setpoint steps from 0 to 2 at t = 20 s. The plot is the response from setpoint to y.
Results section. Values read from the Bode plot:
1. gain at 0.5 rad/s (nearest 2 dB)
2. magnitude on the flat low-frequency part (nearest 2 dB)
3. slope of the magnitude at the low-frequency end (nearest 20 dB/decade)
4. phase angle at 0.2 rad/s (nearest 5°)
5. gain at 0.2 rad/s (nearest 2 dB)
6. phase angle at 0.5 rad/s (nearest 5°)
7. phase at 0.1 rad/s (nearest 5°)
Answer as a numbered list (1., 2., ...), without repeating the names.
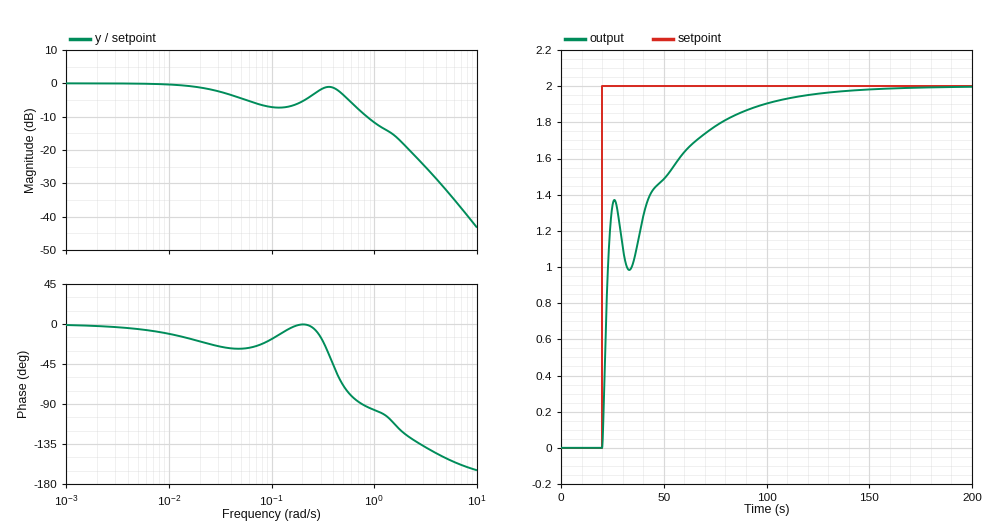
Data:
1. -4 dB
2. 0 dB
3. 0 dB/decade
4. 0°
5. -6 dB
6. -70°
7. -15°
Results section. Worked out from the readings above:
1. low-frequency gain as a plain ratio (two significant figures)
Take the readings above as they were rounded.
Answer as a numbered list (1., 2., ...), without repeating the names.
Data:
1. 1.0
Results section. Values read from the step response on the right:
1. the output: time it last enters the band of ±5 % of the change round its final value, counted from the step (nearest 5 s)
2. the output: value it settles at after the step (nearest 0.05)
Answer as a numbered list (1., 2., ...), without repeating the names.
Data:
1. 80 s
2. 2.00
